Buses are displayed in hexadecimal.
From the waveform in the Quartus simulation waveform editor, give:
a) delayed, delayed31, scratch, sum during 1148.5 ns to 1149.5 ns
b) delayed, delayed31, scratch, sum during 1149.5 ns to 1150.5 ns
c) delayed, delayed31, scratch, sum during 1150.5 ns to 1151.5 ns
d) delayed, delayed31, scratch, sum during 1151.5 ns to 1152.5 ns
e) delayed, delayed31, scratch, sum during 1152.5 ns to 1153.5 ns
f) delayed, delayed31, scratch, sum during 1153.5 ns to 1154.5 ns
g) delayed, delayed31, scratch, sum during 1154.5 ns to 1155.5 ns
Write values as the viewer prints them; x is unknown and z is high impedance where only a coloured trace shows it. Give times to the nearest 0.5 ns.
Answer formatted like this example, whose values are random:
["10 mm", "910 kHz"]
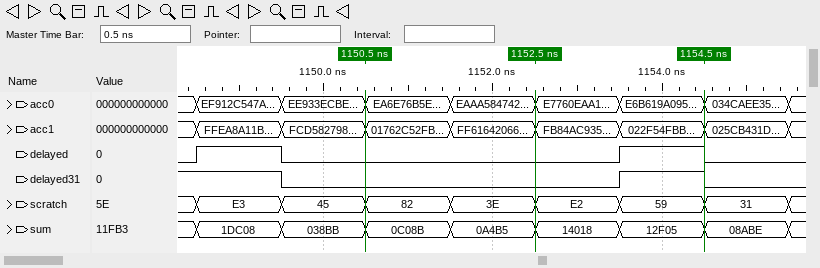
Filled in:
["delayed=1, delayed31=1, scratch=E3, sum=1DC08", "delayed=0, delayed31=0, scratch=45, sum=038BB", "delayed=0, delayed31=0, scratch=82, sum=0C08B", "delayed=0, delayed31=0, scratch=3E, sum=0A4B5", "delayed=0, delayed31=0, scratch=E2, sum=14018", "delayed=1, delayed31=1, scratch=59, sum=12F05", "delayed=0, delayed31=0, scratch=31, sum=08ABE"]
